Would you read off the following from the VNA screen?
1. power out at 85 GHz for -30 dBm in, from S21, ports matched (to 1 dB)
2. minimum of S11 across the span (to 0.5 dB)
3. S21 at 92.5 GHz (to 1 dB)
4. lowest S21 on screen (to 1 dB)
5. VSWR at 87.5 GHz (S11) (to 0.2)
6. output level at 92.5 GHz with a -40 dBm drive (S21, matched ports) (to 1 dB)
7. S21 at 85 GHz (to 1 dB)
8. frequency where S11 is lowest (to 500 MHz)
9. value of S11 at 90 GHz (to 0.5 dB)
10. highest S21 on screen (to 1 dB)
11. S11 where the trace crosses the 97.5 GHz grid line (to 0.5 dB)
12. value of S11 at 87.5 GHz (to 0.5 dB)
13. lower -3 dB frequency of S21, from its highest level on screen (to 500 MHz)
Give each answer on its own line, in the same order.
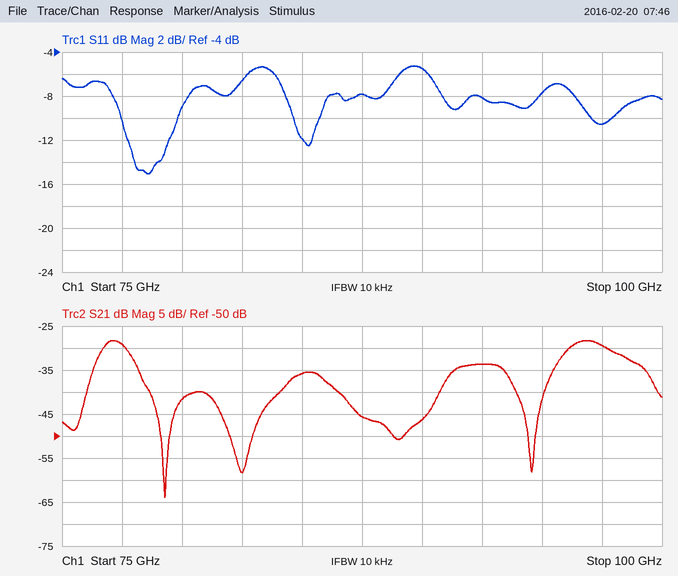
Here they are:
-66 dBm
-15.0 dB
-34 dB
-64 dB
2.4
-74 dBm
-36 dB
78.5 GHz
-5.5 dB
-28 dB
-10.5 dB
-8.0 dB
76.5 GHz
